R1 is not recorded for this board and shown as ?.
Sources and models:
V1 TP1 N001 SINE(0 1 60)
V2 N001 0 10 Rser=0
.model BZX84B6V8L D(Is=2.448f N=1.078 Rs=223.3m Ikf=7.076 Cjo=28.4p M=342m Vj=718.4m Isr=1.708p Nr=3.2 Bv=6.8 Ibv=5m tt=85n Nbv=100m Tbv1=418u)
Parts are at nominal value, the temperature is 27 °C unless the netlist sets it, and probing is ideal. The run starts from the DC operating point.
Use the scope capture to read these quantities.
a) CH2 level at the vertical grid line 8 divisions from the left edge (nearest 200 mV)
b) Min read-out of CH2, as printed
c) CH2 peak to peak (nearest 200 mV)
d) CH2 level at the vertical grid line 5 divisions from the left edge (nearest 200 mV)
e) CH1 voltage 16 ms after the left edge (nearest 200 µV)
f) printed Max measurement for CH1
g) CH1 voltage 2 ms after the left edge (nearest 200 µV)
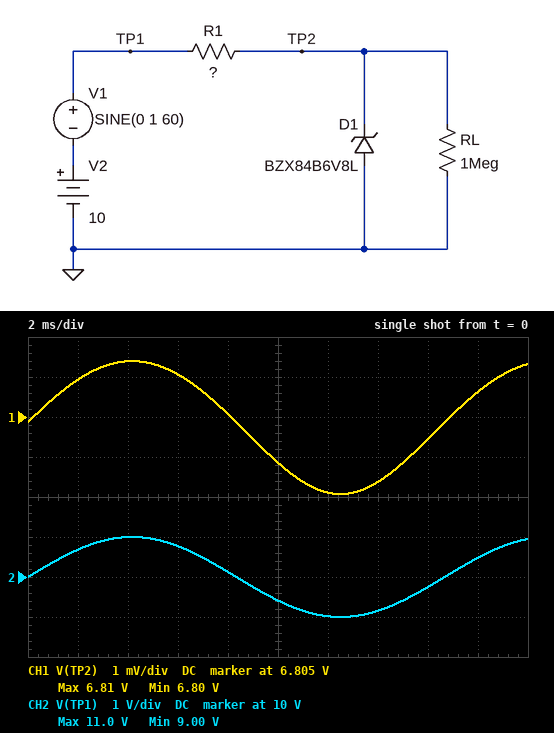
9.8 V
9.00 V
2.0 V
9.4 V
6.8044 V
6.81 V
6.8060 V
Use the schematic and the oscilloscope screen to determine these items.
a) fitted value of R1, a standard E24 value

270 Ω
